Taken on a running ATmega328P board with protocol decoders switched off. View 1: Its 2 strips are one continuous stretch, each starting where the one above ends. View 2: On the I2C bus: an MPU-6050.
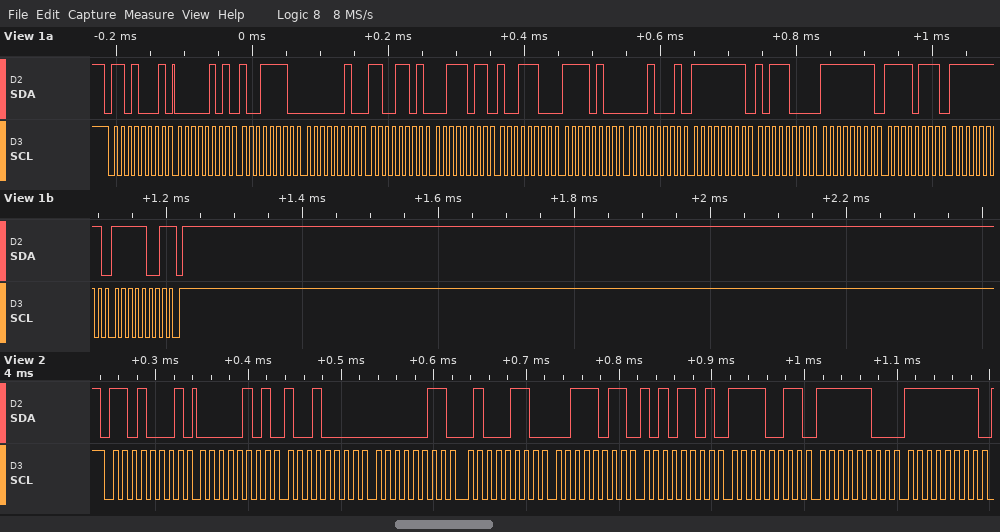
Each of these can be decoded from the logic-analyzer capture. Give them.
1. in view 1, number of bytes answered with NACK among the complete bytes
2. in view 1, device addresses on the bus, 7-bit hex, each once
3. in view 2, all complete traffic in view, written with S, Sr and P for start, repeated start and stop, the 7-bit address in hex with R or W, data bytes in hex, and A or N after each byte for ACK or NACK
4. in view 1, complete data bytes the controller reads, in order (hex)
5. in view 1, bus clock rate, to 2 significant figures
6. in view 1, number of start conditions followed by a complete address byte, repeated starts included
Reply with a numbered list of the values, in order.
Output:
1. 1
2. 0x68
3. S 68R A 05 A 90 A 03 A 46 A 3B A AD A F3 A FC A FF A
4. 05 9E 02 CD 3B 9C F4 11 FF B8 FF F7 FF F9
5. 100 kHz
6. 1
